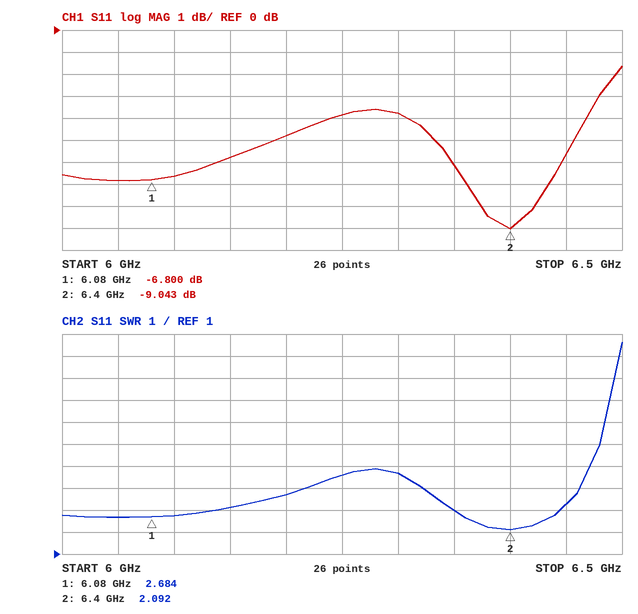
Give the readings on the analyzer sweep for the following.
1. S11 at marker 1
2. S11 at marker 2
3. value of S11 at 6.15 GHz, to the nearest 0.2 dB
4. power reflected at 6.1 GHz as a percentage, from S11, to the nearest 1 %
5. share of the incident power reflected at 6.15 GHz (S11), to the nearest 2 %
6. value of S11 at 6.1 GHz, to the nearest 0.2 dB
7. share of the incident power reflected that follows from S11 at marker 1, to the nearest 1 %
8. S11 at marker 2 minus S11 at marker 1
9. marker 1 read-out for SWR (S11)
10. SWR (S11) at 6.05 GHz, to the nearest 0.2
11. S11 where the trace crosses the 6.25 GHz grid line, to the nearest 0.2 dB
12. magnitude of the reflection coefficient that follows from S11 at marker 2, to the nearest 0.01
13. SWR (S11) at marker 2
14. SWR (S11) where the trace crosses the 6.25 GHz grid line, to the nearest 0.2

-6.800 dB
-9.043 dB
-5.8 dB
22 %
26 %
-6.6 dB
21 %
-2.243 dB
2.684
2.6
-3.8 dB
0.35
2.092
4.6
